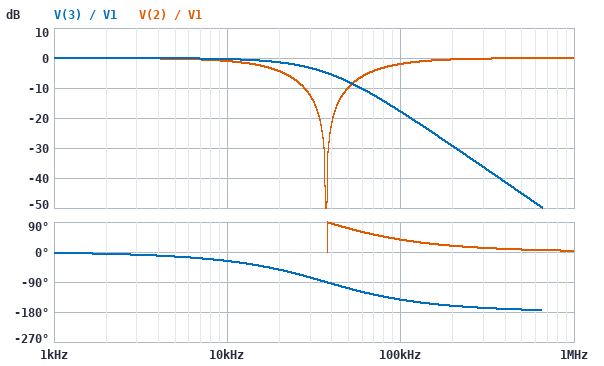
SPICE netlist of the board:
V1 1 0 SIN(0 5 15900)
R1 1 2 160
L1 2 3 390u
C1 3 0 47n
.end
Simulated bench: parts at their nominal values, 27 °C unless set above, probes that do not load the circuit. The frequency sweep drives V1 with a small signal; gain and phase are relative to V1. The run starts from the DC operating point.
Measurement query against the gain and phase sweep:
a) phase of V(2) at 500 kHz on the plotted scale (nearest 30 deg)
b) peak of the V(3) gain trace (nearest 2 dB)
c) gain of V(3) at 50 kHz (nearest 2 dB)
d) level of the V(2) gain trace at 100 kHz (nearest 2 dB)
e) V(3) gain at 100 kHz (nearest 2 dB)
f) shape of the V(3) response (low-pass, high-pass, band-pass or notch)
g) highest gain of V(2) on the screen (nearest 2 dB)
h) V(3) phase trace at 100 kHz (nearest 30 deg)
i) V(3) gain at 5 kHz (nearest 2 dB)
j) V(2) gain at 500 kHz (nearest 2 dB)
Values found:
0 deg
0 dB
-8 dB
-2 dB
-18 dB
low-pass
0 dB
-150 deg
0 dB
0 dB
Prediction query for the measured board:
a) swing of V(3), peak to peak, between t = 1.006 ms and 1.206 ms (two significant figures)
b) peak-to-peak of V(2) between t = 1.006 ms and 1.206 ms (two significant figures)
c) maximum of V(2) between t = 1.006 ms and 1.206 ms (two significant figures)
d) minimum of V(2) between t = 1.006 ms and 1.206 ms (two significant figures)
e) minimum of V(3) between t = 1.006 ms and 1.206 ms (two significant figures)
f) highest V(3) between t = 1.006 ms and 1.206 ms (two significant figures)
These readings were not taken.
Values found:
9.0 V
7.4 V
3.7 V
-3.7 V
-4.5 V
4.5 V
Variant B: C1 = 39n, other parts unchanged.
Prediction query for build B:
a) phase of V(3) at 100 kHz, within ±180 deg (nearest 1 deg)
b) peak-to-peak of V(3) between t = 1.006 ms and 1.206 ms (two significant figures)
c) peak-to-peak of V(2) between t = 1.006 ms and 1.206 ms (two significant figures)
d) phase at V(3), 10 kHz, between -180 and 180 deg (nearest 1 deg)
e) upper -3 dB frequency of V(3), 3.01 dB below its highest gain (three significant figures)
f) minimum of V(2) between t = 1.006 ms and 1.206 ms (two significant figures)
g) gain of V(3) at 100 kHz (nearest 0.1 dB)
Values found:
-142 deg
9.5 V
8.1 V
-23 deg
35.5 kHz
-4.0 V
-16.1 dB
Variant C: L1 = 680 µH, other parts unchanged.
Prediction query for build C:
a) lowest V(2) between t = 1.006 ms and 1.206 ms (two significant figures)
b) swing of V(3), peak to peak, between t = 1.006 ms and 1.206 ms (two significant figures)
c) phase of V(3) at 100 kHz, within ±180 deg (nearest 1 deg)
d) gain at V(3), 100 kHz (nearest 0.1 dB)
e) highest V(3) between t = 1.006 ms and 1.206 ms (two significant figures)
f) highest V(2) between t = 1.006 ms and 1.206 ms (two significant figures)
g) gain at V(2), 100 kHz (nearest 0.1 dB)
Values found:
-3.4 V
9.9 V
-158 deg
-22.0 dB
4.9 V
3.4 V
-0.7 dB
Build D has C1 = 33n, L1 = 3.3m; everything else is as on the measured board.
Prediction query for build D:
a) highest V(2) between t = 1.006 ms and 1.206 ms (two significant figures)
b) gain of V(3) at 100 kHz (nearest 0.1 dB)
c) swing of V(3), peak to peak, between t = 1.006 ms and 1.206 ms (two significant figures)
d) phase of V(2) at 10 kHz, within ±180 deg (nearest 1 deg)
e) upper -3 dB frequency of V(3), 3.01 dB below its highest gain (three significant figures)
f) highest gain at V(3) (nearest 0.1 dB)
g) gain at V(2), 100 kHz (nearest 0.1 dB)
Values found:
810 mV
-32.5 dB
19 V
-30 deg
17.8 kHz
6.2 dB
0 dB
